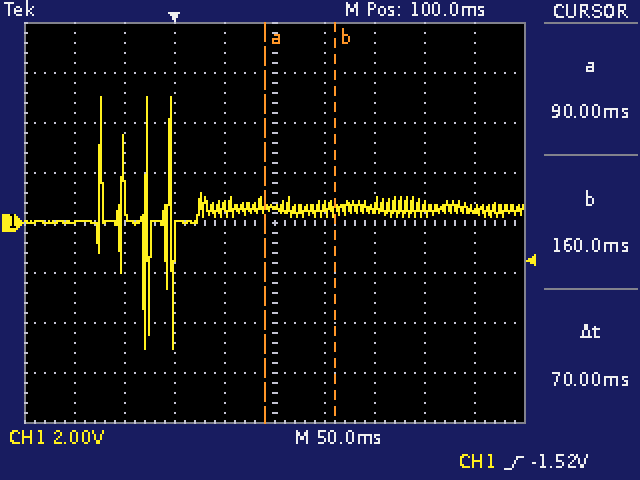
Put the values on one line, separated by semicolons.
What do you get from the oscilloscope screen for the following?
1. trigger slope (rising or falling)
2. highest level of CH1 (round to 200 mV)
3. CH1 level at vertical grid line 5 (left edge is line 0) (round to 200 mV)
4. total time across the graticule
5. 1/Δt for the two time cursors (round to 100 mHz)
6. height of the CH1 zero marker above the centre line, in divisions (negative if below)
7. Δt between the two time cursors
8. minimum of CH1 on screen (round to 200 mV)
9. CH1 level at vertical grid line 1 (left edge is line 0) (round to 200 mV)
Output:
rising; 5.0 V; 600 mV; 500 ms; 14.3 Hz; 0.0 div; 70 ms; -5.0 V; 0.0 V
